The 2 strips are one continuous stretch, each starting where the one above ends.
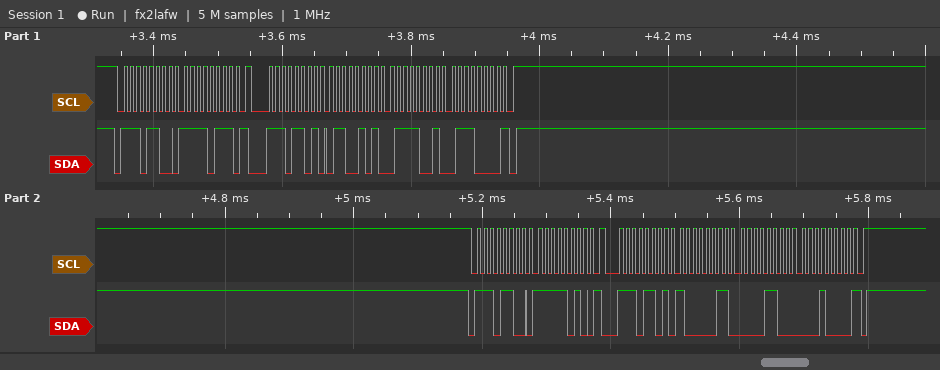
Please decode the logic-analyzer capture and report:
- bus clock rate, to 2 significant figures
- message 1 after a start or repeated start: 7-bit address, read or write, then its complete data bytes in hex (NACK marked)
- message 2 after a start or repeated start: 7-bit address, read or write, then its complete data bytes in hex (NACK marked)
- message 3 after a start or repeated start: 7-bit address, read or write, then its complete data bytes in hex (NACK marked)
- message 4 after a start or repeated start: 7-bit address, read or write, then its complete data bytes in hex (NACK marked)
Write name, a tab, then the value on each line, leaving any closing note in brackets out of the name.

bus clock rate, to 2 significant figures	100 kHz
message 1 after a start or repeated start: 7-bit address, read or write, then its complete data bytes in hex	0x76 write: F7
message 2 after a start or repeated start: 7-bit address, read or write, then its complete data bytes in hex	0x76 read: 65 79 70 NACK
message 3 after a start or repeated start: 7-bit address, read or write, then its complete data bytes in hex	0x76 write: FA
message 4 after a start or repeated start: 7-bit address, read or write, then its complete data bytes in hex	0x76 read: 83 0C 10 NACK
